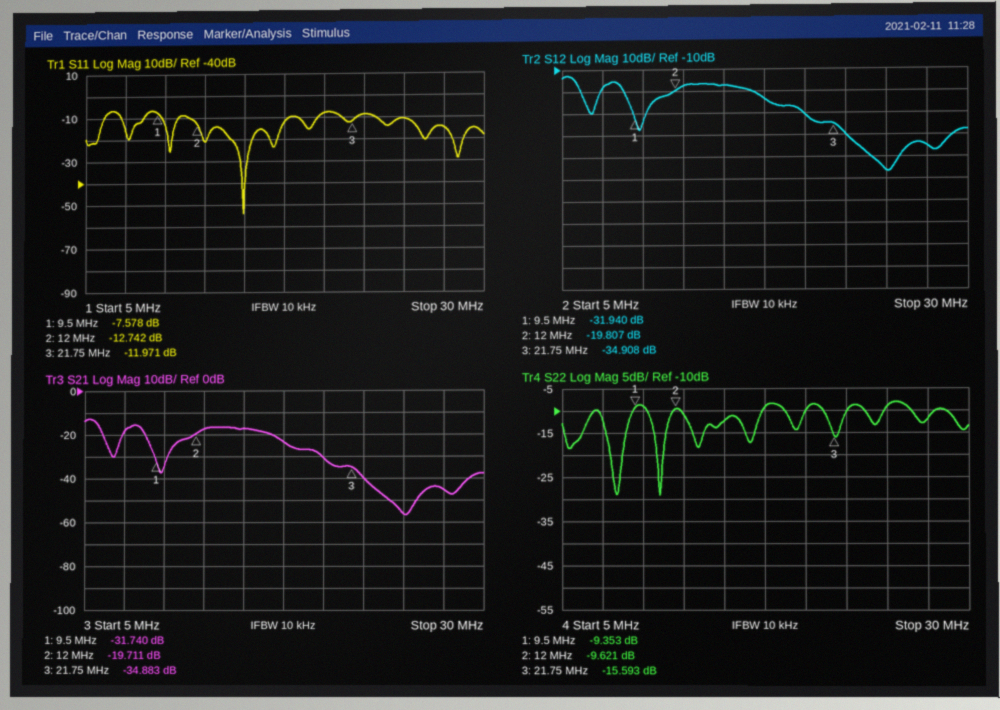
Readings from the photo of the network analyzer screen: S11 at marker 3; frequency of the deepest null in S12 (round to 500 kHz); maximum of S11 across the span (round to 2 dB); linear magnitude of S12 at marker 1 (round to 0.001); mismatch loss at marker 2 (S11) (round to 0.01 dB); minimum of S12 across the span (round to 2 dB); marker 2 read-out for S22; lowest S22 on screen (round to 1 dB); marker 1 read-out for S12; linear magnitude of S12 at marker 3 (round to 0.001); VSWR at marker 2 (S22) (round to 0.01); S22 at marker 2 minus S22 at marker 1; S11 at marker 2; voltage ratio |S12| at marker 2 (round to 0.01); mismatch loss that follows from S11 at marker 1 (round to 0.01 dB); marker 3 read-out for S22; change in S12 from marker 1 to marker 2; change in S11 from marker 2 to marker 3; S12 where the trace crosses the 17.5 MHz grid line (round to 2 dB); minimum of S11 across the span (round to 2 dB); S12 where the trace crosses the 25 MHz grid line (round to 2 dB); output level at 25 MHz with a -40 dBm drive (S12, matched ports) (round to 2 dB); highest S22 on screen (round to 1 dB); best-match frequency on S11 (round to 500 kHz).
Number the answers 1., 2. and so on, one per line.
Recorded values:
1. -11.971 dB
2. 25.0 MHz
3. -6 dB
4. 0.025
5. 0.24 dB
6. -56 dB
7. -9.621 dB
8. -29 dB
9. -31.940 dB
10. 0.018
11. 1.99
12. -0.268 dB
13. -12.742 dB
14. 0.10
15. 0.83 dB
16. -15.593 dB
17. 12.133 dB
18. 0.771 dB
19. -24 dB
20. -54 dB
21. -56 dB
22. -96 dBm
23. -8 dB
24. 15.0 MHz
